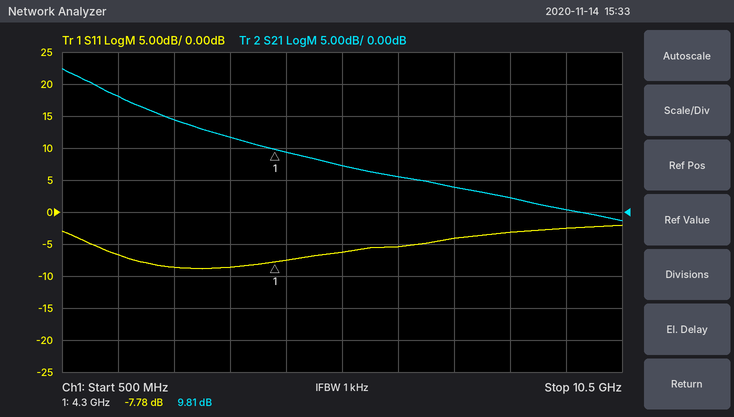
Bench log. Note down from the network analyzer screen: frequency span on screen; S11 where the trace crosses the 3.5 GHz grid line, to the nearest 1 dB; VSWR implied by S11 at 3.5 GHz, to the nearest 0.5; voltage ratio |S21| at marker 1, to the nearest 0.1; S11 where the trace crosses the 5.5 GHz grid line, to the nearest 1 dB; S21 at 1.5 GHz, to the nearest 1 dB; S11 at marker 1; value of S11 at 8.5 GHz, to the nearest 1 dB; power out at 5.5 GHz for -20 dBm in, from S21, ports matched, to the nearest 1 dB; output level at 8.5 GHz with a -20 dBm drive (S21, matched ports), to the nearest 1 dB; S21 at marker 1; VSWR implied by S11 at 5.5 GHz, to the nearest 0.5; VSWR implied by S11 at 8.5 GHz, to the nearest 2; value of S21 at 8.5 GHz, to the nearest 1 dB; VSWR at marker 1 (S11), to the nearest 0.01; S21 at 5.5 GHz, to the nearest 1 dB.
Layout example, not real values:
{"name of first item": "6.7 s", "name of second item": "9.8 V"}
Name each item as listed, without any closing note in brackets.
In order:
{"frequency span on screen": "10 GHz", "S11 where the trace crosses the 3.5 GHz grid line, to the nearest 1 dB": "-9 dB", "VSWR implied by S11 at 3.5 GHz, to the nearest 0.5": "2.0", "voltage ratio |S21| at marker 1, to the nearest 0.1": "3.1", "S11 where the trace crosses the 5.5 GHz grid line, to the nearest 1 dB": "-6 dB", "S21 at 1.5 GHz, to the nearest 1 dB": "18 dB", "S11 at marker 1": "-7.78 dB", "value of S11 at 8.5 GHz, to the nearest 1 dB": "-3 dB", "power out at 5.5 GHz for -20 dBm in, from S21, ports matched, to the nearest 1 dB": "-13 dBm", "output level at 8.5 GHz with a -20 dBm drive (S21, matched ports), to the nearest 1 dB": "-18 dBm", "S21 at marker 1": "9.81 dB", "VSWR implied by S11 at 5.5 GHz, to the nearest 0.5": "3.0", "VSWR implied by S11 at 8.5 GHz, to the nearest 2": "6", "value of S21 at 8.5 GHz, to the nearest 1 dB": "2 dB", "VSWR at marker 1 (S11), to the nearest 0.01": "2.38", "S21 at 5.5 GHz, to the nearest 1 dB": "7 dB"}
